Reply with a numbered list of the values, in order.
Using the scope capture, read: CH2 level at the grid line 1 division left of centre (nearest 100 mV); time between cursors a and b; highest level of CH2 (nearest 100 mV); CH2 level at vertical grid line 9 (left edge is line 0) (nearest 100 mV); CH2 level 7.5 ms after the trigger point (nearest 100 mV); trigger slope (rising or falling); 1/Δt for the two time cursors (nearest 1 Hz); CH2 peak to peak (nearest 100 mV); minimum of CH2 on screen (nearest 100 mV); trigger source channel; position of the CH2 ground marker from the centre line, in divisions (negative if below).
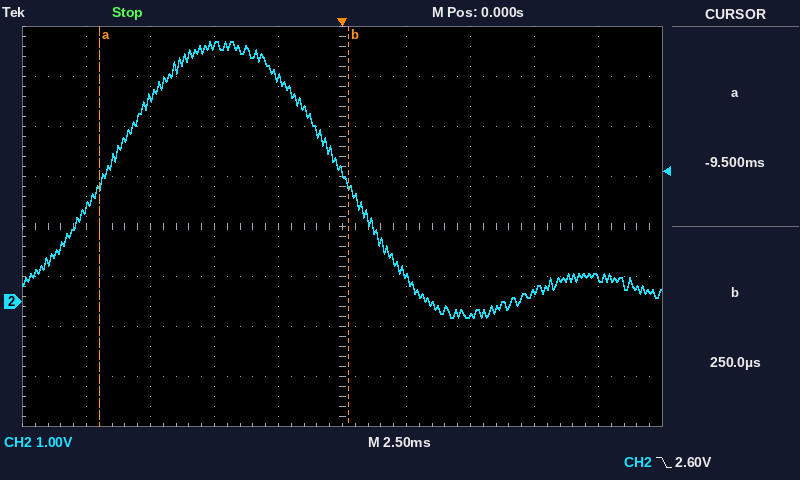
1. 4.5 V
2. 9.75 ms
3. 5.2 V
4. 500 mV
5. 200 mV
6. falling
7. 103 Hz
8. 5.5 V
9. -300 mV
10. CH2
11. -1.5 div
